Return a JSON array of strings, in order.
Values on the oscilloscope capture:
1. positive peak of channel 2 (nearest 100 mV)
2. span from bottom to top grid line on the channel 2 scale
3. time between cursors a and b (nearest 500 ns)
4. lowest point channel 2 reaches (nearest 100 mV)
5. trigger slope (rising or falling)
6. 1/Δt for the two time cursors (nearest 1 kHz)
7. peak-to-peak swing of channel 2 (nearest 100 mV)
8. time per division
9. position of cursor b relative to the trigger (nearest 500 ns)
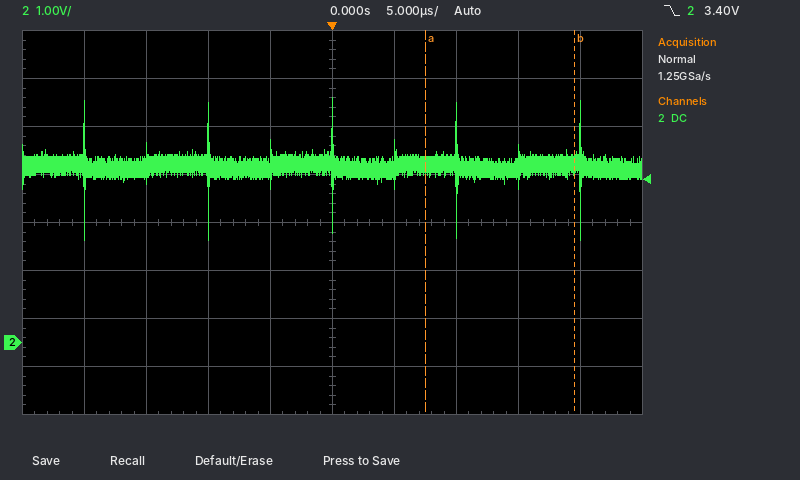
["5.1 V", "8 V", "12.0 µs", "2.1 V", "falling", "83 kHz", "3.0 V", "5 µs", "+19.5 µs"]
